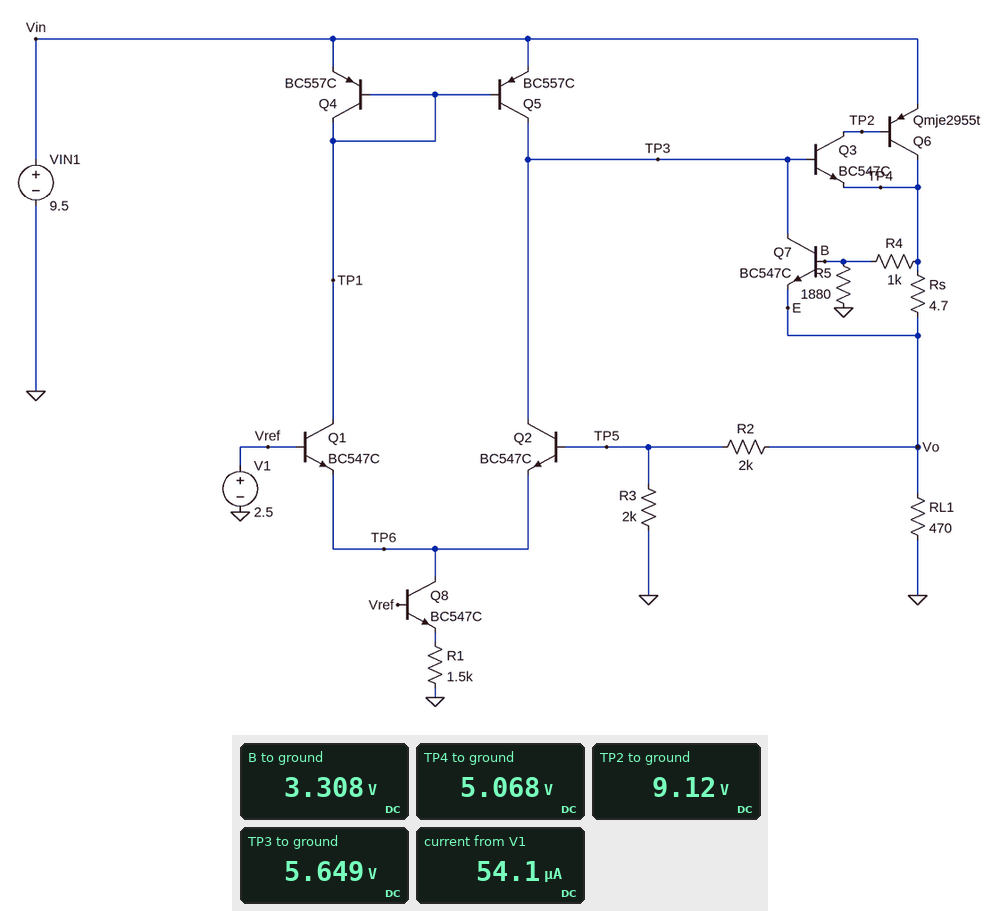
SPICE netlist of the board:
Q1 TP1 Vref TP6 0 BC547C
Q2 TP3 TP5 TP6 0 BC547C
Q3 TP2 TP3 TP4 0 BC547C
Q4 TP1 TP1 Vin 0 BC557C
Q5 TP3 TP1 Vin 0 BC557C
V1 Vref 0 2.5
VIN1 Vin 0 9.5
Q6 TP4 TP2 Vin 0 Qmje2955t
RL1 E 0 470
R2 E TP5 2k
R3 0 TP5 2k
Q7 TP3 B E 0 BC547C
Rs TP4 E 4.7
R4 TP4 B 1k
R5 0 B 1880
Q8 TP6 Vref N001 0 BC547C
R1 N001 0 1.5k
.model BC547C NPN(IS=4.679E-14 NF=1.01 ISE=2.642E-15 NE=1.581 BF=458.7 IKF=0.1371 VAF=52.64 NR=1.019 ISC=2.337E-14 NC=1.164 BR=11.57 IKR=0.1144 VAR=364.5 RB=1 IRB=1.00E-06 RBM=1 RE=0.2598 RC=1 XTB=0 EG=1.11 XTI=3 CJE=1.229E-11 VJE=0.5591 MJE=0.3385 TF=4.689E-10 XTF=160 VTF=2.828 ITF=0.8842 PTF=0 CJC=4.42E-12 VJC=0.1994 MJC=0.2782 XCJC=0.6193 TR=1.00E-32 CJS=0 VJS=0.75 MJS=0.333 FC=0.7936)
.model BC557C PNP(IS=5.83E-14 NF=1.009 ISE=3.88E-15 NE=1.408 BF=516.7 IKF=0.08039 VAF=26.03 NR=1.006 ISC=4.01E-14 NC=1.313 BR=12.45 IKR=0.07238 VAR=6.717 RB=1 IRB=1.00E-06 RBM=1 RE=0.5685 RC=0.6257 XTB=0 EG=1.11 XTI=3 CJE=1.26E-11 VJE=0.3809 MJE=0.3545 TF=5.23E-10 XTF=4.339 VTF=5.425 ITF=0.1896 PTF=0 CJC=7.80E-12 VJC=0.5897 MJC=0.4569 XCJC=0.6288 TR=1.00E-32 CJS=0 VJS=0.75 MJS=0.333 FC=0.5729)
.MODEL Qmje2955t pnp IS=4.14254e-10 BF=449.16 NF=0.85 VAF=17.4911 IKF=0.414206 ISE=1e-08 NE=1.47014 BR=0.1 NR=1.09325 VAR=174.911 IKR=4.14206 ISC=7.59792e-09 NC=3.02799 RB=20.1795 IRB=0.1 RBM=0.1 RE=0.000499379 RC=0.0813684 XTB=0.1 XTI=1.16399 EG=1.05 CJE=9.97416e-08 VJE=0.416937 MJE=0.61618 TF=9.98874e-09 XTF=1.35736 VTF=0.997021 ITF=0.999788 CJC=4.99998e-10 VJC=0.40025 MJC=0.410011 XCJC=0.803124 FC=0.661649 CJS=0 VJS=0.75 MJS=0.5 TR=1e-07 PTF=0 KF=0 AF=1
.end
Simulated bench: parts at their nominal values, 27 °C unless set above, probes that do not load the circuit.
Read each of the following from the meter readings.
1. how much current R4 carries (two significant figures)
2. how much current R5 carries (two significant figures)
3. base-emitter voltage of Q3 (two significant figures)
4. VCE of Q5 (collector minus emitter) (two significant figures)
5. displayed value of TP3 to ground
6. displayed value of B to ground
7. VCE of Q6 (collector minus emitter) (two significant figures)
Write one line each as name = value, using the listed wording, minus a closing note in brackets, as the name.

how much current R4 carries = 1.8 mA
how much current R5 carries = 1.8 mA
base-emitter voltage of Q3 = 580 mV
VCE of Q5 (collector minus emitter) = -3.9 V
displayed value of TP3 to ground = 5.649 V
displayed value of B to ground = 3.308 V
VCE of Q6 (collector minus emitter) = -4.4 V
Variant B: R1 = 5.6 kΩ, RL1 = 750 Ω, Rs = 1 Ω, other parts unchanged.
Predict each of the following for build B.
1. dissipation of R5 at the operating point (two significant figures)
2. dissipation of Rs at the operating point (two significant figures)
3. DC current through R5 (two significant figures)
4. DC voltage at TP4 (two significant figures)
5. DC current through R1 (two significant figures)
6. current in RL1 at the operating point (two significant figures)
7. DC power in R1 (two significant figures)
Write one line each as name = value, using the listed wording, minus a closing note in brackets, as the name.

dissipation of R5 at the operating point = 5.7 mW
dissipation of Rs at the operating point = 63 µW
DC current through R5 = 1.7 mA
DC voltage at TP4 = 5.0 V
DC current through R1 = 340 µA
current in RL1 at the operating point = 6.7 mA
DC power in R1 = 640 µW
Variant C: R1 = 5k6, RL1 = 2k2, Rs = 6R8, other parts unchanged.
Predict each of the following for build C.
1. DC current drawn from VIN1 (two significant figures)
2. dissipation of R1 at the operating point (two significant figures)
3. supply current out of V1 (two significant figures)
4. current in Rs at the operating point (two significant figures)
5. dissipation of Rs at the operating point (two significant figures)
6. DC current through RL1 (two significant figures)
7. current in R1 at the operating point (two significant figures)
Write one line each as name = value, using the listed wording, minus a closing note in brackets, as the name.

DC current drawn from VIN1 = 5.6 mA
dissipation of R1 at the operating point = 640 µW
supply current out of V1 = 15 µA
current in Rs at the operating point = 3.5 mA
dissipation of Rs at the operating point = 85 µW
DC current through RL1 = 2.3 mA
current in R1 at the operating point = 340 µA
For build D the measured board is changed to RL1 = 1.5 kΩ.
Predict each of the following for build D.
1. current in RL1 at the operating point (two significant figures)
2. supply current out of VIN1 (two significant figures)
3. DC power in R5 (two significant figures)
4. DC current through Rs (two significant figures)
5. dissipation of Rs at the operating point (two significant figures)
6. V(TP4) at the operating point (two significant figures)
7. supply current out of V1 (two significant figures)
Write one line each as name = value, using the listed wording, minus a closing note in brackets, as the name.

current in RL1 at the operating point = 3.3 mA
supply current out of VIN1 = 7.5 mA
DC power in R5 = 5.7 mW
DC current through Rs = 4.6 mA
dissipation of Rs at the operating point = 99 µW
V(TP4) at the operating point = 5.0 V
supply current out of V1 = 54 µA
